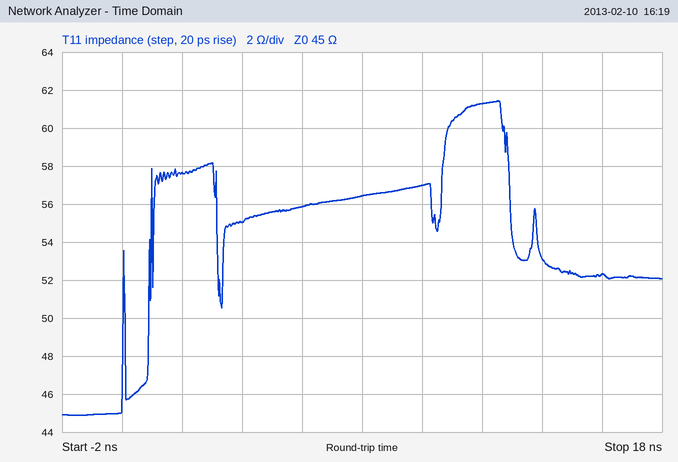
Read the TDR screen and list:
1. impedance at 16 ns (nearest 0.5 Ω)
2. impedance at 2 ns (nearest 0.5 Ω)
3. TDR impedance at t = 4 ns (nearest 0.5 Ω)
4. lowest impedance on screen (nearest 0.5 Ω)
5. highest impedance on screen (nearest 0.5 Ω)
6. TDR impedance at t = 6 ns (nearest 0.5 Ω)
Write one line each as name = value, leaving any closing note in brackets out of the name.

impedance at 16 ns = 52.5 Ω
impedance at 2 ns = 57.5 Ω
TDR impedance at t = 4 ns = 55.0 Ω
lowest impedance on screen = 45.0 Ω
highest impedance on screen = 61.5 Ω
TDR impedance at t = 6 ns = 56.0 Ω
